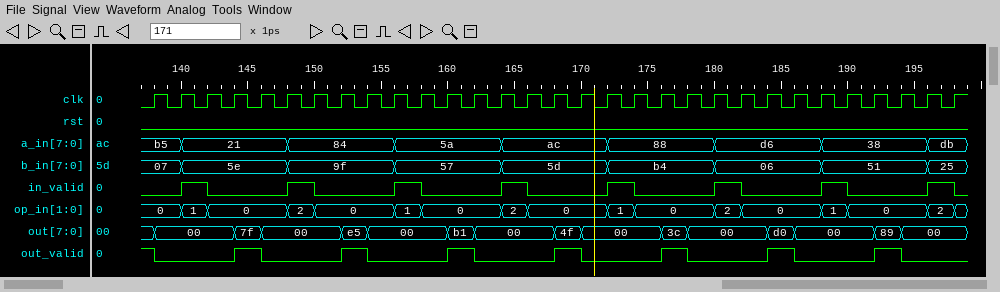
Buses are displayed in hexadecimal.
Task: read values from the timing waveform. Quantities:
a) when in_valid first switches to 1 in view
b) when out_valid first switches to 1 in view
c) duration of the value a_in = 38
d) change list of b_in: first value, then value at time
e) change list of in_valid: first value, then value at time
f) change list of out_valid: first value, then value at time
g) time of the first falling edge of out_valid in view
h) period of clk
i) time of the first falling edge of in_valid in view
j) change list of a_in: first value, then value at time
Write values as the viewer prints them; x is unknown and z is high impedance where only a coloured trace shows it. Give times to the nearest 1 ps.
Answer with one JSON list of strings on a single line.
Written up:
["140 ps", "144 ps", "8 ps", "07, 5e at 140 ps, 9f at 148 ps, 57 at 156 ps, 5d at 164 ps, b4 at 172 ps, 06 at 180 ps, 51 at 188 ps, 25 at 196 ps", "0, 1 at 140 ps, 0 at 142 ps, 1 at 148 ps, 0 at 150 ps, 1 at 156 ps, 0 at 158 ps, 1 at 164 ps, 0 at 166 ps, 1 at 172 ps, 0 at 174 ps, 1 at 180 ps, 0 at 182 ps, 1 at 188 ps, 0 at 190 ps, 1 at 196 ps, 0 at 198 ps", "1, 0 at 138 ps, 1 at 144 ps, 0 at 146 ps, 1 at 152 ps, 0 at 154 ps, 1 at 160 ps, 0 at 162 ps, 1 at 168 ps, 0 at 170 ps, 1 at 176 ps, 0 at 178 ps, 1 at 184 ps, 0 at 186 ps, 1 at 192 ps, 0 at 194 ps", "138 ps", "2 ps", "142 ps", "b5, 21 at 140 ps, 84 at 148 ps, 5a at 156 ps, ac at 164 ps, 88 at 172 ps, d6 at 180 ps, 38 at 188 ps, db at 196 ps"]
